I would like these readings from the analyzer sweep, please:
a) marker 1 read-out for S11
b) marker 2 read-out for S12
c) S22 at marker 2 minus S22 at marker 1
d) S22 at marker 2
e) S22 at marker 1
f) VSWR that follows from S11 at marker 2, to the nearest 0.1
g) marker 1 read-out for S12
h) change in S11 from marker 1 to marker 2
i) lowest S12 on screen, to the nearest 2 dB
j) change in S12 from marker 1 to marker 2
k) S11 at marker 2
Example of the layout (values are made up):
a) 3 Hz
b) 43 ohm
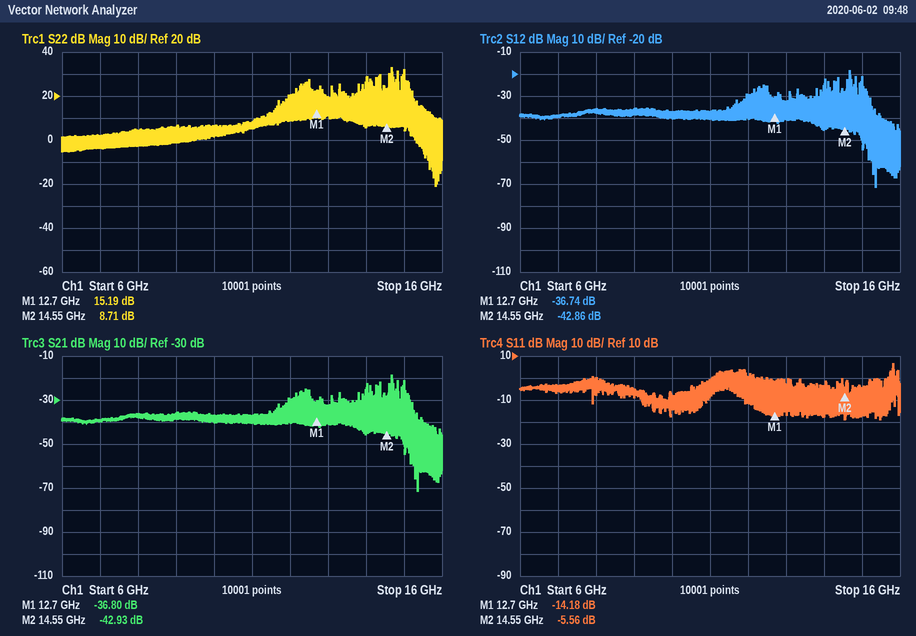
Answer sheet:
a) -14.18 dB
b) -42.86 dB
c) -6.48 dB
d) 8.71 dB
e) 15.19 dB
f) 3.2
g) -36.74 dB
h) 8.62 dB
i) -72 dB
j) -6.12 dB
k) -5.56 dB
